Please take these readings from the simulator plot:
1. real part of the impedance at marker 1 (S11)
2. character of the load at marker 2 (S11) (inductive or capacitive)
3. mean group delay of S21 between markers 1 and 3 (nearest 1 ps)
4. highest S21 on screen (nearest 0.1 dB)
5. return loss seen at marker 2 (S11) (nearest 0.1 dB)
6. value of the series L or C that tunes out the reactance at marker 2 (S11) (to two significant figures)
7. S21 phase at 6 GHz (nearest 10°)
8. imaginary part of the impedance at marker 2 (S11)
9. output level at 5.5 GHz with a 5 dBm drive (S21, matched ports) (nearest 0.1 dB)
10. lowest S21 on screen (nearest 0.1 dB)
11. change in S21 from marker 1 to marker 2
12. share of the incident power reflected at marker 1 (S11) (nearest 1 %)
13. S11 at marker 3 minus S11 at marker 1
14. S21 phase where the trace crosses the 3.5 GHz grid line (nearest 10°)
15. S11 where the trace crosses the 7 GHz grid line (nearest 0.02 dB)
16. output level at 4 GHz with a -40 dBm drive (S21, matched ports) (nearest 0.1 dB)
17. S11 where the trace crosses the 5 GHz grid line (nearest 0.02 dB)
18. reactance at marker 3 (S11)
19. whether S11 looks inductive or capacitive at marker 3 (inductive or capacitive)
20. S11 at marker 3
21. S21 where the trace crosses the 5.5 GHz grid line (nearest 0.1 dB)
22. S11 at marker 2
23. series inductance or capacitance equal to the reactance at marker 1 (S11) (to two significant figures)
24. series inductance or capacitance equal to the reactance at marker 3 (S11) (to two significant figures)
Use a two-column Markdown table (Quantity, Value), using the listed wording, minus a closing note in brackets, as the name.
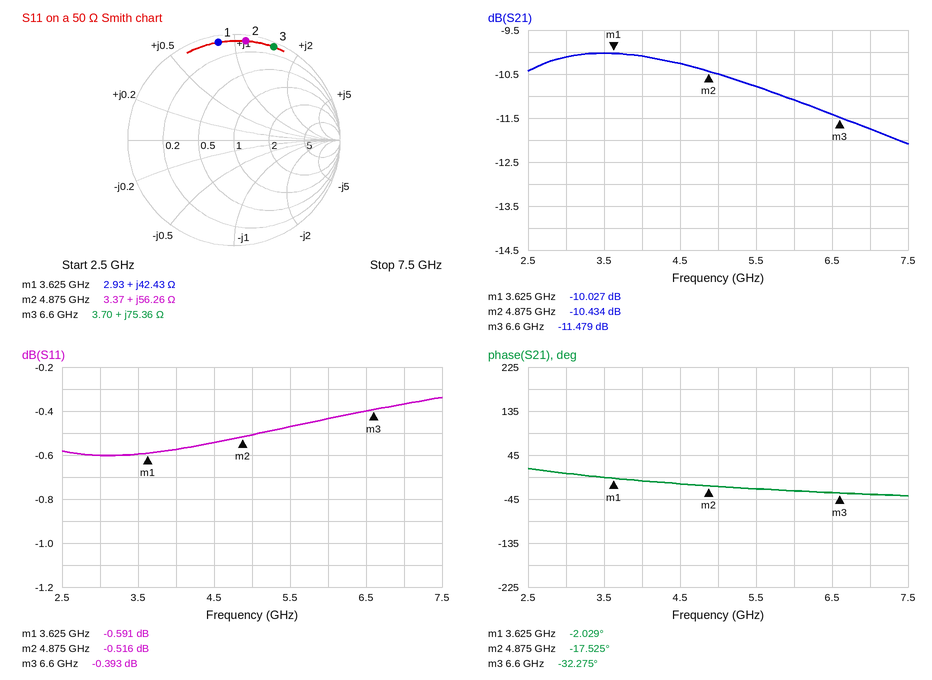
| Quantity | Value |
|---|---|
| real part of the impedance at marker 1 | 2.93 Ω |
| character of the load at marker 2 (S11) | inductive |
| mean group delay of S21 between markers 1 and 3 | 28 ps |
| highest S21 on screen | -10.0 dB |
| return loss seen at marker 2 (S11) | 0.5 dB |
| value of the series L or C that tunes out the reactance at marker 2 (S11) | 580 fF |
| S21 phase at 6 GHz | -30° |
| imaginary part of the impedance at marker 2 | +56.26 Ω |
| output level at 5.5 GHz with a 5 dBm drive (S21, matched ports) | -5.8 dBm |
| lowest S21 on screen | -12.1 dB |
| change in S21 from marker 1 to marker 2 | -0.407 dB |
| share of the incident power reflected at marker 1 (S11) | 87 % |
| S11 at marker 3 minus S11 at marker 1 | 0.198 dB |
| S21 phase where the trace crosses the 3.5 GHz grid line | 0° |
| S11 where the trace crosses the 7 GHz grid line | -0.36 dB |
| output level at 4 GHz with a -40 dBm drive (S21, matched ports) | -50.1 dBm |
| S11 where the trace crosses the 5 GHz grid line | -0.50 dB |
| reactance at marker 3 | +75.36 Ω |
| whether S11 looks inductive or capacitive at marker 3 | inductive |
| S11 at marker 3 | -0.393 dB |
| S21 where the trace crosses the 5.5 GHz grid line | -10.8 dB |
| S11 at marker 2 | -0.516 dB |
| series inductance or capacitance equal to the reactance at marker 1 (S11) | 1.9 nH |
| series inductance or capacitance equal to the reactance at marker 3 (S11) | 1.8 nH |
